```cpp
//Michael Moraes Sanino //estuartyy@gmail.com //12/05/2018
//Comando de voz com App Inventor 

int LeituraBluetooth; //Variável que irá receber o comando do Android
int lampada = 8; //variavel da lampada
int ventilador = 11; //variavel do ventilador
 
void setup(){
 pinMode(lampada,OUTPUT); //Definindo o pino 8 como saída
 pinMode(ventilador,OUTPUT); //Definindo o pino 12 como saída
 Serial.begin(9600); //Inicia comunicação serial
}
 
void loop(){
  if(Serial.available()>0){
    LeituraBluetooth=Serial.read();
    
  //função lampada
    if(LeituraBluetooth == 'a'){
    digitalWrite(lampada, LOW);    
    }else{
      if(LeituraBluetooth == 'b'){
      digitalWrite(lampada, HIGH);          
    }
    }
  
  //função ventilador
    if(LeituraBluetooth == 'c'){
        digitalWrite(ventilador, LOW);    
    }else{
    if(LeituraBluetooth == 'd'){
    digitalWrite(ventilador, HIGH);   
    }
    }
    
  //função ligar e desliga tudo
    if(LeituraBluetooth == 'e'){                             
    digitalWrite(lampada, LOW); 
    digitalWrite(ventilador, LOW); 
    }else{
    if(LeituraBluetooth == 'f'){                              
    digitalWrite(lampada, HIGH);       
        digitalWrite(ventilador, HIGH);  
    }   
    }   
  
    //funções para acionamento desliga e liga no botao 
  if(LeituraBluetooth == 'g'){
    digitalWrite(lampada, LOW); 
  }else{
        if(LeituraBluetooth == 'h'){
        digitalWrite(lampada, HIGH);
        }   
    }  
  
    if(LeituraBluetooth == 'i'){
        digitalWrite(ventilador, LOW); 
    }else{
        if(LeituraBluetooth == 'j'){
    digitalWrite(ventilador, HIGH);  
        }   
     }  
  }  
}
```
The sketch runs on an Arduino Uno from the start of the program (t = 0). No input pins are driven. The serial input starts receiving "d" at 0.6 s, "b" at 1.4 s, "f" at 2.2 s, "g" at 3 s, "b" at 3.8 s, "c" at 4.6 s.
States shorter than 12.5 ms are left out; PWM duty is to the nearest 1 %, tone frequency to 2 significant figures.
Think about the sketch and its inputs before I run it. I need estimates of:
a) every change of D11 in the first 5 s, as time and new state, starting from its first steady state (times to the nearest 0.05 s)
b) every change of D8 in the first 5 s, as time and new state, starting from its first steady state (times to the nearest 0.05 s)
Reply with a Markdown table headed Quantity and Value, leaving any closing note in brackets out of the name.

| Quantity | Value |
|---|---|
| every change of D11 in the first 5 s, as time and new state, starting from its first steady state | 0 s low; 0.6 s high; 4.6 s low |
| every change of D8 in the first 5 s, as time and new state, starting from its first steady state | 0 s low; 1.4 s high; 3 s low; 3.8 s high |
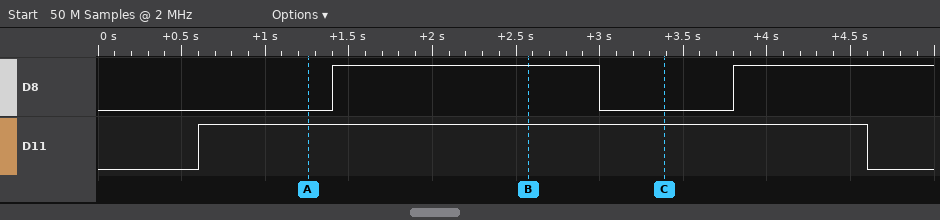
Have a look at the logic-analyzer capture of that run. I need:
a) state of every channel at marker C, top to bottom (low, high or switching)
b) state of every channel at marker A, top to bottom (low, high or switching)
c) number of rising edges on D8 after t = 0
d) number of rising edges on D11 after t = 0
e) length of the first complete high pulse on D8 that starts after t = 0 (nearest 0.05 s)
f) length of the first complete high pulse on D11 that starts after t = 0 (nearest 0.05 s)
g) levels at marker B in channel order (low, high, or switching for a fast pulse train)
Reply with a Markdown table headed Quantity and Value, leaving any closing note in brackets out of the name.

| Quantity | Value |
|---|---|
| state of every channel at marker C, top to bottom | D8 low, D11 high |
| state of every channel at marker A, top to bottom | D8 low, D11 high |
| number of rising edges on D8 after t = 0 | 2 |
| number of rising edges on D11 after t = 0 | 1 |
| length of the first complete high pulse on D8 that starts after t = 0 | 1.60 s |
| length of the first complete high pulse on D11 that starts after t = 0 | 4.00 s |
| levels at marker B in channel order | D8 high, D11 high |
